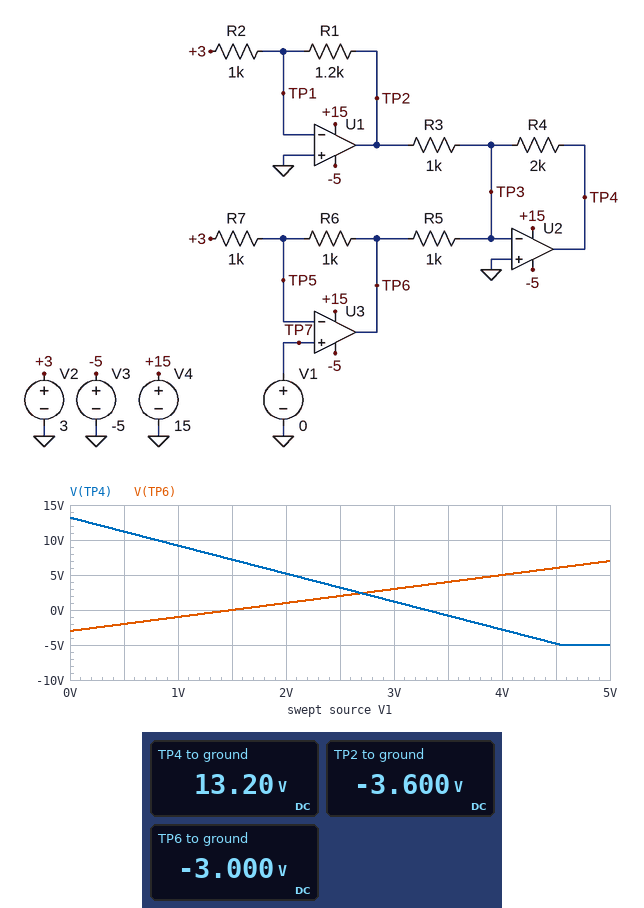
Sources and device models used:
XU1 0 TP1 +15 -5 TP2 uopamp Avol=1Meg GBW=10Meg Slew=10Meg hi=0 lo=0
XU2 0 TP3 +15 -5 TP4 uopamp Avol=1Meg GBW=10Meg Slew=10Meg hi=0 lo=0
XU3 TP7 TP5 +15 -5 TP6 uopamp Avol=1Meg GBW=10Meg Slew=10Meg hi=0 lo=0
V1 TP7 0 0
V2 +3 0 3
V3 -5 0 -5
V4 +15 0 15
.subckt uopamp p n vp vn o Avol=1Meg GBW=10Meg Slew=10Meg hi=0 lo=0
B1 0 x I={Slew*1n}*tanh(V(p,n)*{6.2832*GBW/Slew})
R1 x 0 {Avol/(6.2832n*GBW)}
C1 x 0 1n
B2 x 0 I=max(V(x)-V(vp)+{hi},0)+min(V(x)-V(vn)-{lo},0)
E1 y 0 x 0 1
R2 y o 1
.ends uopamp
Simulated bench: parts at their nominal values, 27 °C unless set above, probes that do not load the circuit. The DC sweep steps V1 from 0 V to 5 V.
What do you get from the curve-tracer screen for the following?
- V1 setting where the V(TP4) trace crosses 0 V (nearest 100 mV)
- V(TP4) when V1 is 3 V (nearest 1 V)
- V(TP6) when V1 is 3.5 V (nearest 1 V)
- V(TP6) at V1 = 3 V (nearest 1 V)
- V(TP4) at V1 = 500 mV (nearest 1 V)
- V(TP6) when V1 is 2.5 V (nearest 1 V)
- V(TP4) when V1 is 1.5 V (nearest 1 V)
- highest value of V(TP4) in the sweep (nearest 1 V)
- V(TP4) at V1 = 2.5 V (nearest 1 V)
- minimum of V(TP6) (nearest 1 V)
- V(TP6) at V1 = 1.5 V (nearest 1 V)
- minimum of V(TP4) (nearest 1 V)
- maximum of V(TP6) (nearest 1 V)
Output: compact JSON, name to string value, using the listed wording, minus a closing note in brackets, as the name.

{"V1 setting where the V(TP4) trace crosses 0 V": "3.3 V", "V(TP4) when V1 is 3 V": "1 V", "V(TP6) when V1 is 3.5 V": "4 V", "V(TP6) at V1 = 3 V": "3 V", "V(TP4) at V1 = 500 mV": "11 V", "V(TP6) when V1 is 2.5 V": "2 V", "V(TP4) when V1 is 1.5 V": "7 V", "highest value of V(TP4) in the sweep": "13 V", "V(TP4) at V1 = 2.5 V": "3 V", "minimum of V(TP6)": "-3 V", "V(TP6) at V1 = 1.5 V": "0 V", "minimum of V(TP4)": "-5 V", "maximum of V(TP6)": "7 V"}
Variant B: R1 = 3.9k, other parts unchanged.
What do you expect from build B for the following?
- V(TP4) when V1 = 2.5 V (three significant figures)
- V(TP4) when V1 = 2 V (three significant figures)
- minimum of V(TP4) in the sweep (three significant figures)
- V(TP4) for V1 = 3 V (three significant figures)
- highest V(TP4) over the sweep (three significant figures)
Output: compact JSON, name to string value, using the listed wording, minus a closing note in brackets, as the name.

{"V(TP4) when V1 = 2.5 V": "6.01 V", "V(TP4) when V1 = 2 V": "8.01 V", "minimum of V(TP4) in the sweep": "-3.99 V", "V(TP4) for V1 = 3 V": "4.01 V", "highest V(TP4) over the sweep": "15.0 V"}
